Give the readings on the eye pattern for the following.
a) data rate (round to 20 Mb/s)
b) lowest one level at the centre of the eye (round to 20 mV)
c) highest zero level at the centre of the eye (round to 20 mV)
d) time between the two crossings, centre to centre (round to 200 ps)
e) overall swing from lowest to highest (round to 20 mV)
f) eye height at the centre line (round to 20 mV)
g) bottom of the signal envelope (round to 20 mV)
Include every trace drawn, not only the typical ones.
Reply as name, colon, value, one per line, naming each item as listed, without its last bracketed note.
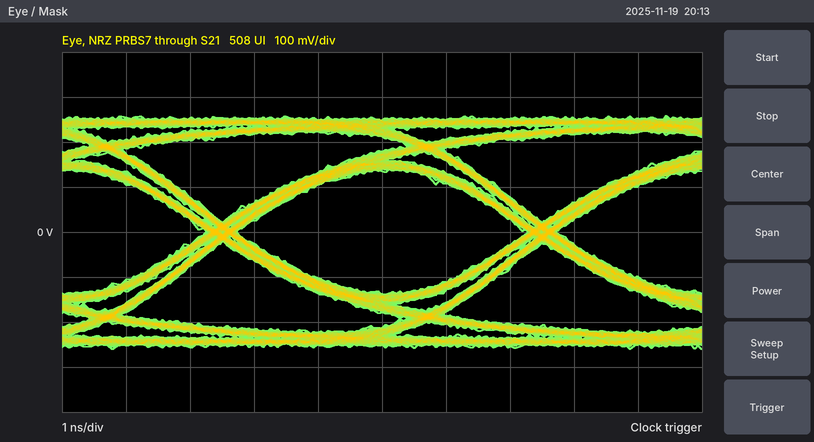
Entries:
data rate: 200 Mb/s
lowest one level at the centre of the eye: 140 mV
highest zero level at the centre of the eye: -140 mV
time between the two crossings, centre to centre: 5.0 ns
overall swing from lowest to highest: 520 mV
eye height at the centre line: 280 mV
bottom of the signal envelope: -260 mV
